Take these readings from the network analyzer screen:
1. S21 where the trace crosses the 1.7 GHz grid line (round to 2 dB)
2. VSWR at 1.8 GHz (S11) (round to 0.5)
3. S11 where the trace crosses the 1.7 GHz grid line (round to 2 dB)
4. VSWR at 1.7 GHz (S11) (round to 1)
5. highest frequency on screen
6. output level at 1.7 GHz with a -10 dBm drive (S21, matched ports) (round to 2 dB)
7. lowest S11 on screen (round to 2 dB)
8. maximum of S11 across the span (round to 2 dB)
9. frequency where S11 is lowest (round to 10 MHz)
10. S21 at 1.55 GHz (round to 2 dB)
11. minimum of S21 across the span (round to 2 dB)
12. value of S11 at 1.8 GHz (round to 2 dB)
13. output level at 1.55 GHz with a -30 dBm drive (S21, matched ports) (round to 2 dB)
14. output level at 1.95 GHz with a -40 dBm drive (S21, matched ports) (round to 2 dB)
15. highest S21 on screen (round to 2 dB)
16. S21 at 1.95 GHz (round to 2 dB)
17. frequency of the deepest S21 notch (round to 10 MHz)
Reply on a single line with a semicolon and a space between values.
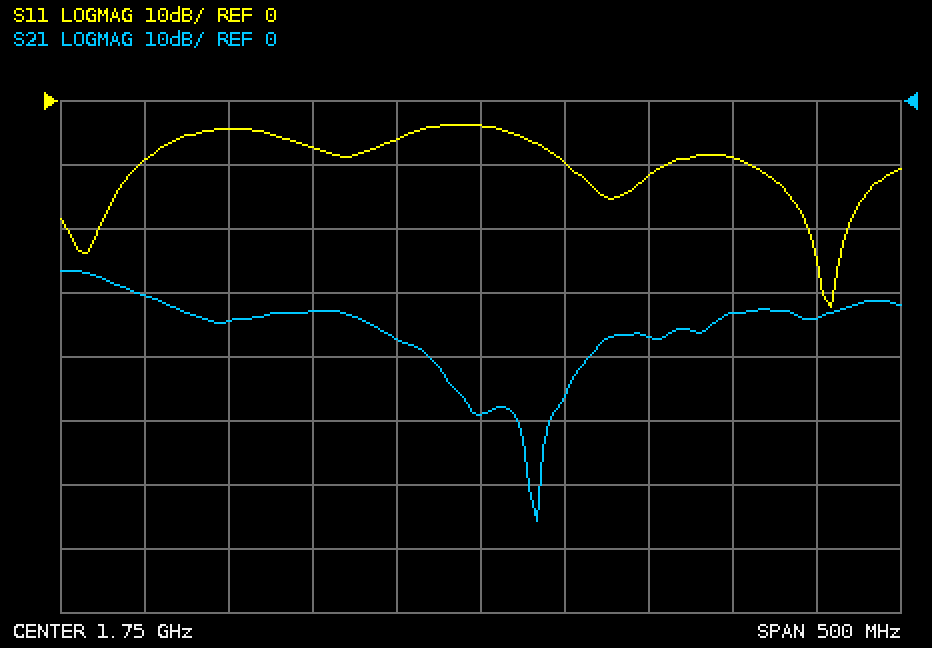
-38 dB; 2.0; -6 dB; 3; 2 GHz; -48 dBm; -32 dB; -4 dB; 1.96 GHz; -30 dB; -66 dB; -10 dB; -60 dBm; -74 dBm; -26 dB; -34 dB; 1.78 GHz
